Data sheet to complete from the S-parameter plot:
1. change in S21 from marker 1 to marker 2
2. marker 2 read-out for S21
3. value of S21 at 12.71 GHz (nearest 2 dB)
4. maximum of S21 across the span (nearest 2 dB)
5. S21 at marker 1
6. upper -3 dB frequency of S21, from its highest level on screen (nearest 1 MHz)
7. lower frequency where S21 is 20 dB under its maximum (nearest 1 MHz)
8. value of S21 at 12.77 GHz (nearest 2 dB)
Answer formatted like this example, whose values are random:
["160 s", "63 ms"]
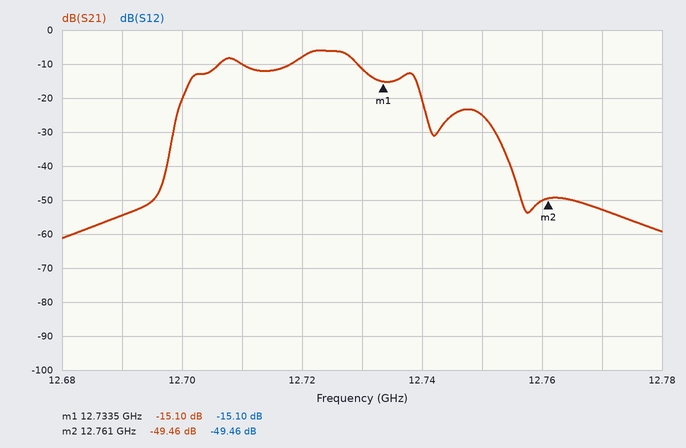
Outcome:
["-34.36 dB", "-49.46 dB", "-10 dB", "-6 dB", "-15.10 dB", "12.729 GHz", "12.699 GHz", "-52 dB"]
